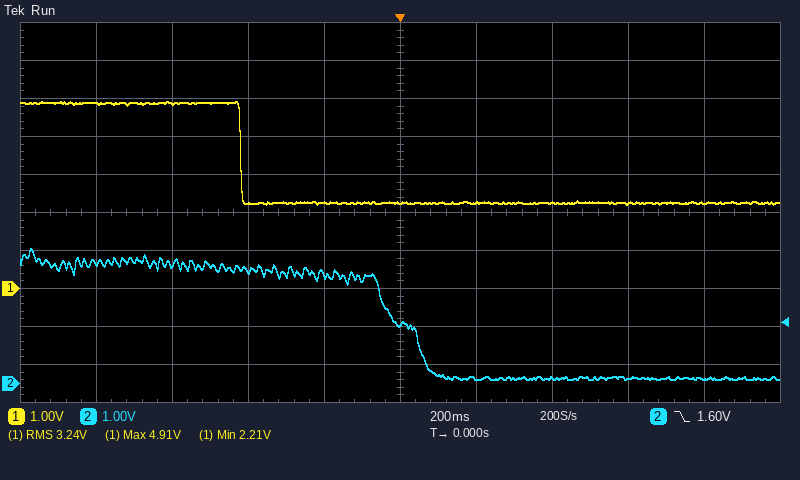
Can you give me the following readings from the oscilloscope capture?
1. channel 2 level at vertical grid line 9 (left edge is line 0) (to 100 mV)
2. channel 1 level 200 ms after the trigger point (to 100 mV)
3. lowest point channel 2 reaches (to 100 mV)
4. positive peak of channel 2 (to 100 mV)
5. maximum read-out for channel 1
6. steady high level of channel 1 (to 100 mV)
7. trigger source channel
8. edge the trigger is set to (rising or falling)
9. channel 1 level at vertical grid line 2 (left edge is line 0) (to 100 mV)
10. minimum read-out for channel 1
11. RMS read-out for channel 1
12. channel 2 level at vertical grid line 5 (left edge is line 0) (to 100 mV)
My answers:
100 mV
2.3 V
100 mV
3.6 V
4.91 V
4.9 V
channel 2
falling
4.9 V
2.21 V
3.24 V
1.6 V
